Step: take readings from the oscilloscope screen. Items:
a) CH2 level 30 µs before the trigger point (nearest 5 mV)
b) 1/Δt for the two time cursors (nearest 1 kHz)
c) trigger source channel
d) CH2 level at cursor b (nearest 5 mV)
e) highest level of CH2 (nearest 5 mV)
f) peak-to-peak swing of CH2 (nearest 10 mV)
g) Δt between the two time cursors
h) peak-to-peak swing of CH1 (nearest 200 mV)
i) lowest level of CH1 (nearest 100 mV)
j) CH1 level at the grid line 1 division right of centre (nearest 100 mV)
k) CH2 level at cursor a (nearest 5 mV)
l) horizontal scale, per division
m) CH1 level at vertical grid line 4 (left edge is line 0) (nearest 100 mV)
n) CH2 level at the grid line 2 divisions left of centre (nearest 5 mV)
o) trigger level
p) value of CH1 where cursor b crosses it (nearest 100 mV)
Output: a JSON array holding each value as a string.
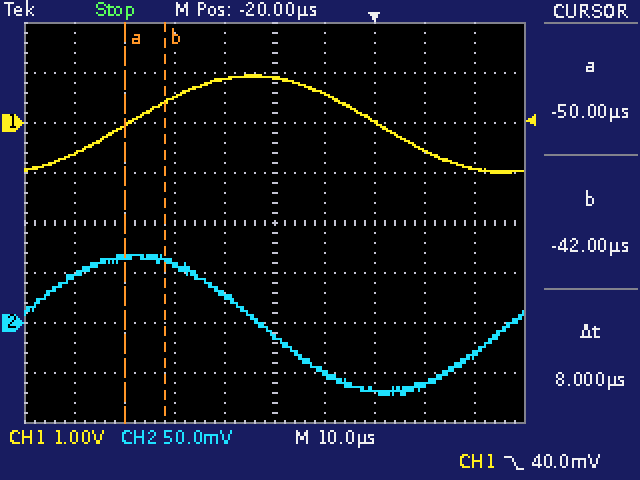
["30 mV", "125 kHz", "CH1", "65 mV", "70 mV", "140 mV", "8 µs", "2.0 V", "-1.0 V", "600 mV", "65 mV", "10 µs", "900 mV", "60 mV", "40.0 mV", "400 mV"]
